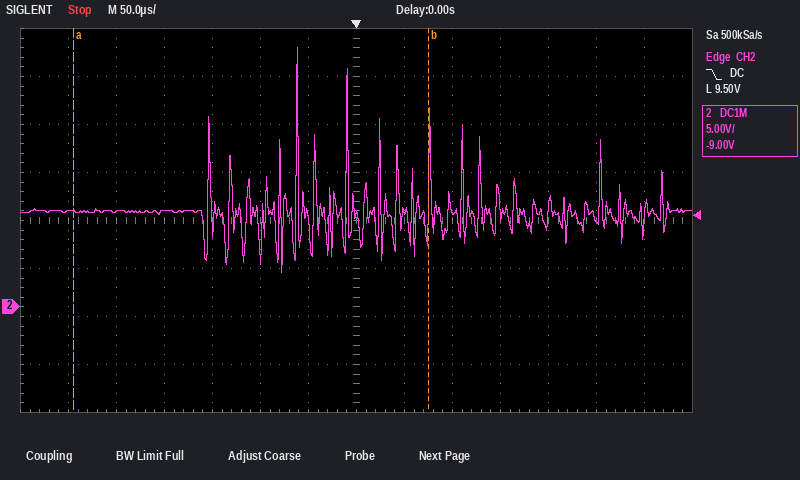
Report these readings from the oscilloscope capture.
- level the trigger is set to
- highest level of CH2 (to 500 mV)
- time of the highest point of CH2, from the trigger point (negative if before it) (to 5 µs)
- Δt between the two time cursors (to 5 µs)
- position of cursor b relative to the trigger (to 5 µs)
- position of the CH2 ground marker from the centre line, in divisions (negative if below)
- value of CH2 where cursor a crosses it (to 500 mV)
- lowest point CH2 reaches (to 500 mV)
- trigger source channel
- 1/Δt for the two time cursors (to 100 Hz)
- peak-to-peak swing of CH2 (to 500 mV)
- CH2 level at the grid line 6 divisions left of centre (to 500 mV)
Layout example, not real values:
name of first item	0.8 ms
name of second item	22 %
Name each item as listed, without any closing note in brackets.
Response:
level the trigger is set to	9.50 V
highest level of CH2	27.0 V
time of the highest point of CH2, from the trigger point (negative if before it)	-60 µs
Δt between the two time cursors	370 µs
position of cursor b relative to the trigger	+75 µs
position of the CH2 ground marker from the centre line, in divisions	-1.8 div
value of CH2 where cursor a crosses it	10.0 V
lowest point CH2 reaches	3.5 V
trigger source channel	CH2
1/Δt for the two time cursors	2.7 kHz
peak-to-peak swing of CH2	23.5 V
CH2 level at the grid line 6 divisions left of centre	10.0 V
